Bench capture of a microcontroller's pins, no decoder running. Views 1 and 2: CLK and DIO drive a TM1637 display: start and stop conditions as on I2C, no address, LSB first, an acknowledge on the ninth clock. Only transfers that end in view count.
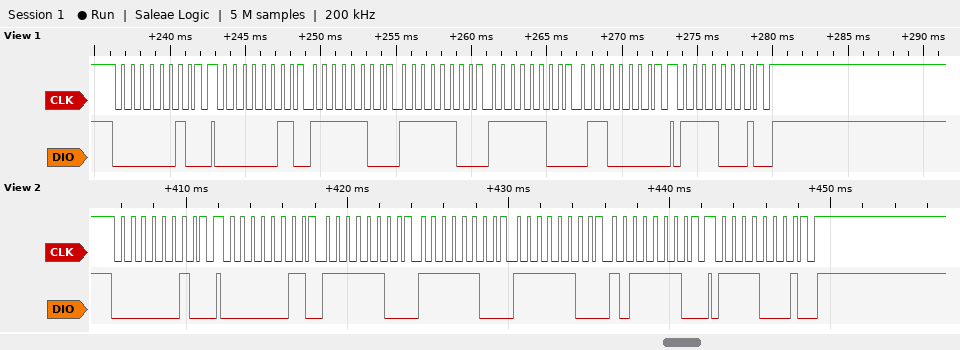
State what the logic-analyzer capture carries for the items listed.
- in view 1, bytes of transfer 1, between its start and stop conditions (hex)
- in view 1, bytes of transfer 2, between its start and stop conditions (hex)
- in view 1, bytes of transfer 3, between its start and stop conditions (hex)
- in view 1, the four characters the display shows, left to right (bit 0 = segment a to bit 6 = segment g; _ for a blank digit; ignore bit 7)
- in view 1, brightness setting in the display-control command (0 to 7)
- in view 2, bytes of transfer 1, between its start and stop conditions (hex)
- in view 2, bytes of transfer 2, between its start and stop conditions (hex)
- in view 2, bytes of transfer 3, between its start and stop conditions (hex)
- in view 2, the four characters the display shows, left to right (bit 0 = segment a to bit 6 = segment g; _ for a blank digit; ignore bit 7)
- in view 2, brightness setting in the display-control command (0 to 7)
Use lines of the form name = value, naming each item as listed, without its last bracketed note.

in view 1, bytes of transfer 1, between its start and stop conditions = 40
in view 1, bytes of transfer 2, between its start and stop conditions = C0 3F 3F 3F 06
in view 1, bytes of transfer 3, between its start and stop conditions = 8F
in view 1, the four characters the display shows, left to right = 0001
in view 1, brightness setting in the display-control command = 7
in view 2, bytes of transfer 1, between its start and stop conditions = 40
in view 2, bytes of transfer 2, between its start and stop conditions = C0 3F 3F 3F 7D
in view 2, bytes of transfer 3, between its start and stop conditions = 8F
in view 2, the four characters the display shows, left to right = 0006
in view 2, brightness setting in the display-control command = 7
